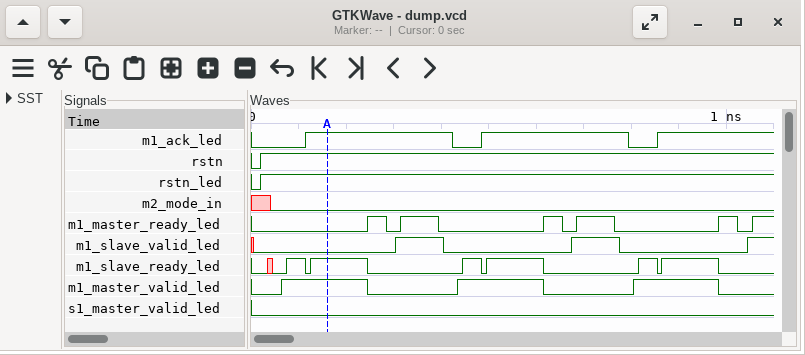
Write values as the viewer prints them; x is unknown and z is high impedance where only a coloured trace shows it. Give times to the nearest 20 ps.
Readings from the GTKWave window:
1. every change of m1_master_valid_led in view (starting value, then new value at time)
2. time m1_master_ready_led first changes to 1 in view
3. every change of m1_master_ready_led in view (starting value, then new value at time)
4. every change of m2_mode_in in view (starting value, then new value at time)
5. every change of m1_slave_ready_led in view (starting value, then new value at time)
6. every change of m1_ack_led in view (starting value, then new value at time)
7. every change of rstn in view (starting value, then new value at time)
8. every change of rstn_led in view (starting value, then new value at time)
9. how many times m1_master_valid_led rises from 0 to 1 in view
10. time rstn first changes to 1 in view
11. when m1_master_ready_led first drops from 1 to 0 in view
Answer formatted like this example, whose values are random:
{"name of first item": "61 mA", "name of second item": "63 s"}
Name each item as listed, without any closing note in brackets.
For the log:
{"every change of m1_master_valid_led in view": "0, 1 at 60 ps, 0 at 240 ps, 1 at 440 ps, 0 at 620 ps, 1 at 800 ps, 0 at 980 ps", "time m1_master_ready_led first changes to 1 in view": "240 ps", "every change of m1_master_ready_led in view": "0, 1 at 240 ps, 0 at 280 ps, 1 at 320 ps, 0 at 400 ps, 1 at 620 ps, 0 at 660 ps, 1 at 680 ps, 0 at 760 ps, 1 at 980 ps, 0 at 1020 ps, 1 at 1060 ps", "every change of m2_mode_in in view": "x, 0 at 40 ps", "every change of m1_slave_ready_led in view": "0, x at 40 ps, 0 at 40 ps, 1 at 80 ps, 0 at 120 ps, 1 at 120 ps, 0 at 240 ps, 1 at 440 ps, 0 at 480 ps, 1 at 500 ps, 0 at 620 ps, 1 at 820 ps, 0 at 860 ps, 1 at 860 ps, 0 at 980 ps", "every change of m1_ack_led in view": "0, 1 at 120 ps, 0 at 420 ps, 1 at 480 ps, 0 at 800 ps, 1 at 860 ps", "every change of rstn in view": "0, 1 at 20 ps", "every change of rstn_led in view": "0, 1 at 20 ps", "how many times m1_master_valid_led rises from 0 to 1 in view": "3", "time rstn first changes to 1 in view": "20 ps", "when m1_master_ready_led first drops from 1 to 0 in view": "280 ps"}
